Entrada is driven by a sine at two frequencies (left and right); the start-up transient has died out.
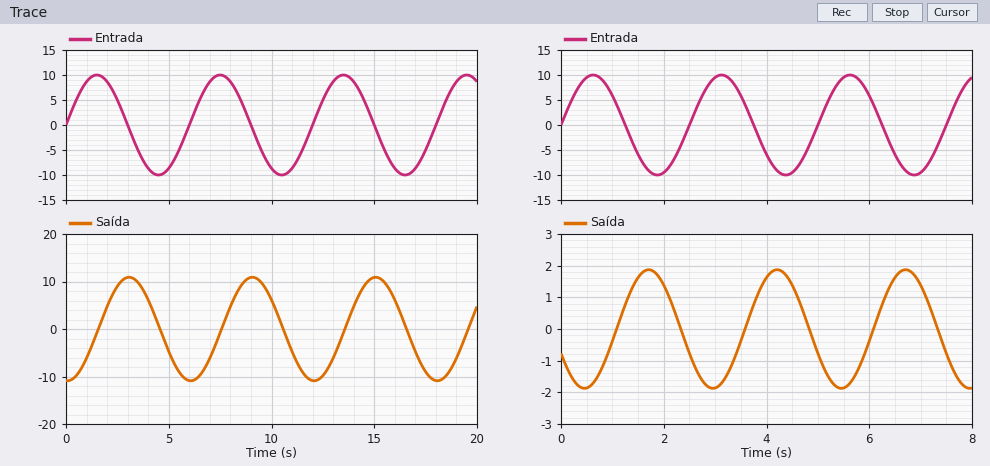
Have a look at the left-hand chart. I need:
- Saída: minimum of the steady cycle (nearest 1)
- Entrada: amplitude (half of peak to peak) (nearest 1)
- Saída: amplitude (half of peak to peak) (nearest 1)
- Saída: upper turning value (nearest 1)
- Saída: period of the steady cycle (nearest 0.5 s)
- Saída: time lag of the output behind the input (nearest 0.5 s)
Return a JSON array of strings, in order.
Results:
["-11", "10", "11", "11", "6.0 s", "1.5 s"]
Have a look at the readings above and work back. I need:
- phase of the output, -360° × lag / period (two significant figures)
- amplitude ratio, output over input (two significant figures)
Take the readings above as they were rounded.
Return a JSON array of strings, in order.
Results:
["-90°", "1.1"]
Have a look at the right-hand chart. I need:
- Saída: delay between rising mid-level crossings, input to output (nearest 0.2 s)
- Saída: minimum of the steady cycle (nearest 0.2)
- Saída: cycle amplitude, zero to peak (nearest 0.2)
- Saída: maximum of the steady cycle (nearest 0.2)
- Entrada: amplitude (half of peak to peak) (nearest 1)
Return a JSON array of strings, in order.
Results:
["1.0 s", "-1.8", "1.8", "1.8", "10"]
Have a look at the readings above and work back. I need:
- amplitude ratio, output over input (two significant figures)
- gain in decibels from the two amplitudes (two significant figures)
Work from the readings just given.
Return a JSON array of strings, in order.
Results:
["0.18", "-15 dB"]
